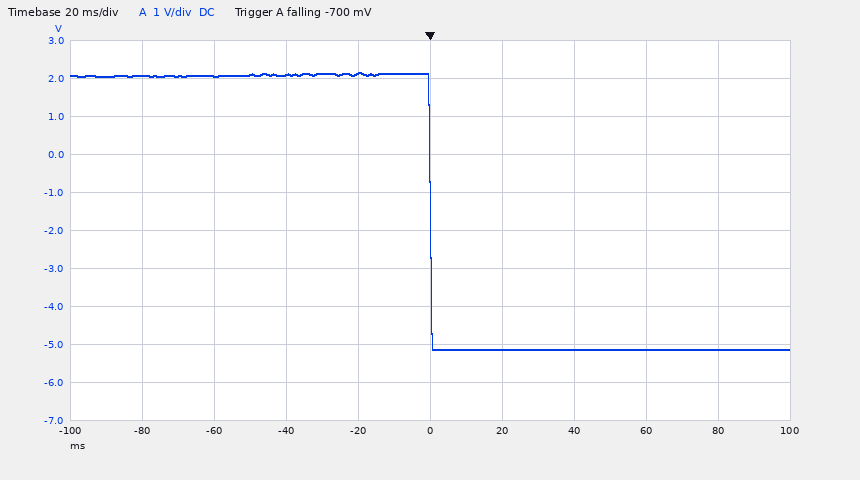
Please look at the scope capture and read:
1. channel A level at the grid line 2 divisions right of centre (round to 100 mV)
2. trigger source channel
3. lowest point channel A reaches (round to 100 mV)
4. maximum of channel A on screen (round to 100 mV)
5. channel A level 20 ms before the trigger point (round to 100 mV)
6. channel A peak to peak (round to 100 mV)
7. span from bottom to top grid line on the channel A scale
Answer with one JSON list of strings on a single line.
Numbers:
["-5.1 V", "channel A", "-5.1 V", "2.2 V", "2.1 V", "7.3 V", "10 V"]
